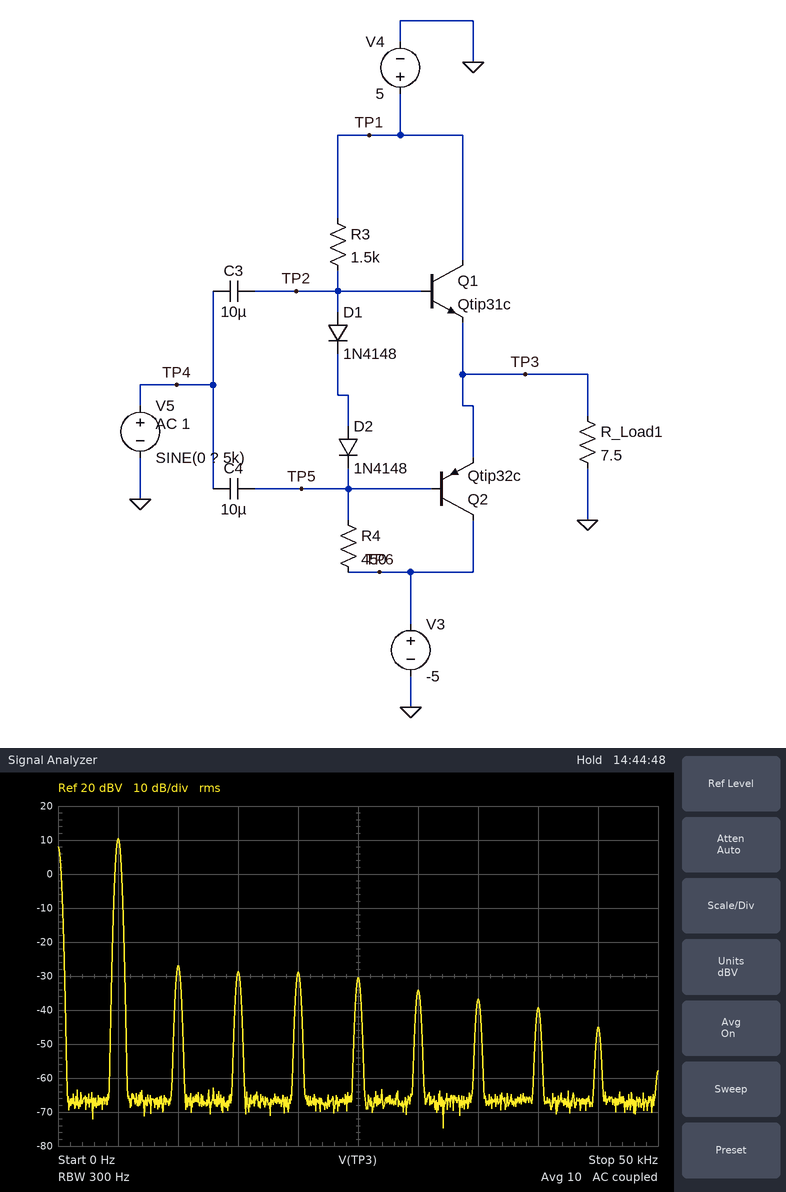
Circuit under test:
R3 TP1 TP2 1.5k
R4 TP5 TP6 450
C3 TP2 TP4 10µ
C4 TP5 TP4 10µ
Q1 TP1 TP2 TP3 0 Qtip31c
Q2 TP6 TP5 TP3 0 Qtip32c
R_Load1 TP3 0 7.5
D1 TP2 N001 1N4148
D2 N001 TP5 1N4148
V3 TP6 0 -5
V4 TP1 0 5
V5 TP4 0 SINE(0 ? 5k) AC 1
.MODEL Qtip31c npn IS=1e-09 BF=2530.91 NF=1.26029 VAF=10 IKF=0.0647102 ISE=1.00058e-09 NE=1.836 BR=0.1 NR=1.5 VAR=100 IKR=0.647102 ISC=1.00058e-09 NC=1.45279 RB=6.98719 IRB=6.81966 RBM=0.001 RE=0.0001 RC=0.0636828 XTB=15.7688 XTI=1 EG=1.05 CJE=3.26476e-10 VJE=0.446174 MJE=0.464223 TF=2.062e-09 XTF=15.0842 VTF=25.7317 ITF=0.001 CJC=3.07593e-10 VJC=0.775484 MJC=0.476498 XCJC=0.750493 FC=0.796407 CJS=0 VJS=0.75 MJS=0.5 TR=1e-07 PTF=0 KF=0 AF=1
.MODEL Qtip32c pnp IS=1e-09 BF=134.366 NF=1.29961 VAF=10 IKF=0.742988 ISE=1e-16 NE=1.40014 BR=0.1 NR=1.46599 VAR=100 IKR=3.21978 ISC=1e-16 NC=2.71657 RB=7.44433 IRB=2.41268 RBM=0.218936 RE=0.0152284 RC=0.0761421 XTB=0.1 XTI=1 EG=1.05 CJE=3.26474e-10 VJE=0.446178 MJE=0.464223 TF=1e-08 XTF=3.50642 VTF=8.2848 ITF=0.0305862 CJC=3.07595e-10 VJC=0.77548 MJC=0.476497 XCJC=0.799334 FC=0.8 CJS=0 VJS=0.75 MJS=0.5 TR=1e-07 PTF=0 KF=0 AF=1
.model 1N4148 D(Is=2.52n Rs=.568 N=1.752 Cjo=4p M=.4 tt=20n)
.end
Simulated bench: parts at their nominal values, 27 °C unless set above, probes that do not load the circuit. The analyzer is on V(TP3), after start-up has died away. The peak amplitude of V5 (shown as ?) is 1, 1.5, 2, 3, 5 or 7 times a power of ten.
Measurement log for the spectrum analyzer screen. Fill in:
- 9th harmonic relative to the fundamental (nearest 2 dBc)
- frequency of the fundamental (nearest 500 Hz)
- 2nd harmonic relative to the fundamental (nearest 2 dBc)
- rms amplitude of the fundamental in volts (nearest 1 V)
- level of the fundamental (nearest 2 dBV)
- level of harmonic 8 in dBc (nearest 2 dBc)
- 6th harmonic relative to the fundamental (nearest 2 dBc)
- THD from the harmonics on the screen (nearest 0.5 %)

-56 dBc
5.0 kHz
-38 dBc
3 V
10 dBV
-50 dBc
-44 dBc
2.5 %
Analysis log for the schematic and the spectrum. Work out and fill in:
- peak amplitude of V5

5 V
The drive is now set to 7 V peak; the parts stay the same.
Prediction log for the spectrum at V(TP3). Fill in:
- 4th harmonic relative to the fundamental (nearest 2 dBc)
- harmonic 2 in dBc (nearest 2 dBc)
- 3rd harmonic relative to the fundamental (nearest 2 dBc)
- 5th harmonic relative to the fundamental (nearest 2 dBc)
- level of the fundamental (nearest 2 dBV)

-32 dBc
-40 dBc
-20 dBc
-22 dBc
10 dBV
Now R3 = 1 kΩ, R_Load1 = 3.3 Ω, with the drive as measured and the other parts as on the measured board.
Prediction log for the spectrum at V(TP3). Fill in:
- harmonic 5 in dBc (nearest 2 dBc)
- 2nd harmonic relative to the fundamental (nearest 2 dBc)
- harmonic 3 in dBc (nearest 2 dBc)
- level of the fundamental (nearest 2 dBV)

-36 dBc
-48 dBc
-36 dBc
10 dBV
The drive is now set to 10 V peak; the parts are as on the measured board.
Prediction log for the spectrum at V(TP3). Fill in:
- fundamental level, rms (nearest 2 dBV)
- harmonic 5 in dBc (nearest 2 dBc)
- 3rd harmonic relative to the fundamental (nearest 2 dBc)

10 dBV
-18 dBc
-12 dBc
